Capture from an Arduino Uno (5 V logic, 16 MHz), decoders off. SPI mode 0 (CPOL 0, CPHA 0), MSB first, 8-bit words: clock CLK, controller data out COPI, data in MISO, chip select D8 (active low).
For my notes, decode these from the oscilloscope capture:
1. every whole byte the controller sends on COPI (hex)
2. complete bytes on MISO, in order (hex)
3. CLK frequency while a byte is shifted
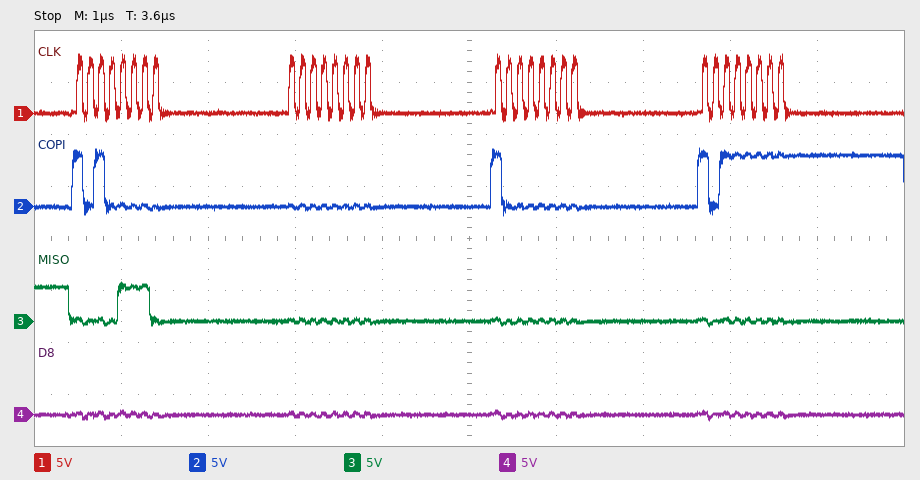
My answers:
A0 00 80 BF
0E 00 00 00
8 MHz
